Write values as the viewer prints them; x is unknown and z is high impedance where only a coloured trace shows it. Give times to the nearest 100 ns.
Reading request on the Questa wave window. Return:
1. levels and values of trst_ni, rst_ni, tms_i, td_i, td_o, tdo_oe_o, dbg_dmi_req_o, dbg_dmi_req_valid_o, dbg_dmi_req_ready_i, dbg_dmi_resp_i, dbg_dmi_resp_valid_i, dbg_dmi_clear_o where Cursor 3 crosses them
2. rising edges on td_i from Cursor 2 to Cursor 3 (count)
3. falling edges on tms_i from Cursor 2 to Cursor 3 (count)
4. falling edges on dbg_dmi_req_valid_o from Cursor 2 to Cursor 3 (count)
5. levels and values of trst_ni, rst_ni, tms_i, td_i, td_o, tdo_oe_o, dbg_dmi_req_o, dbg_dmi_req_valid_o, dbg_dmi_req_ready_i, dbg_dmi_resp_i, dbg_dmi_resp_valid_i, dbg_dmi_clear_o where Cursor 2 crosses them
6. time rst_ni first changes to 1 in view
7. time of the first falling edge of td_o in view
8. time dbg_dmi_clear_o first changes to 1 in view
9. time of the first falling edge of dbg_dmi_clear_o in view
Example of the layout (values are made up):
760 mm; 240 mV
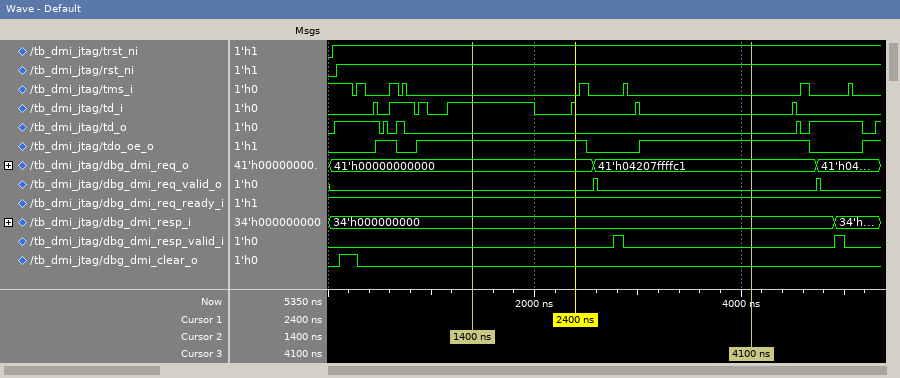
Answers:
trst_ni=1, rst_ni=1, tms_i=0, td_i=0, td_o=0, tdo_oe_o=1, dbg_dmi_req_o=41'h04207ffffc1, dbg_dmi_req_valid_o=0, dbg_dmi_req_ready_i=1, dbg_dmi_resp_i=34'h000000000, dbg_dmi_resp_valid_i=0, dbg_dmi_clear_o=0; 2; 2; 1; trst_ni=1, rst_ni=1, tms_i=0, td_i=1, td_o=0, tdo_oe_o=1, dbg_dmi_req_o=41'h00000000000, dbg_dmi_req_valid_o=0, dbg_dmi_req_ready_i=1, dbg_dmi_resp_i=34'h000000000, dbg_dmi_resp_valid_i=0, dbg_dmi_clear_o=0; 100 ns; 500 ns; 100 ns; 300 ns
